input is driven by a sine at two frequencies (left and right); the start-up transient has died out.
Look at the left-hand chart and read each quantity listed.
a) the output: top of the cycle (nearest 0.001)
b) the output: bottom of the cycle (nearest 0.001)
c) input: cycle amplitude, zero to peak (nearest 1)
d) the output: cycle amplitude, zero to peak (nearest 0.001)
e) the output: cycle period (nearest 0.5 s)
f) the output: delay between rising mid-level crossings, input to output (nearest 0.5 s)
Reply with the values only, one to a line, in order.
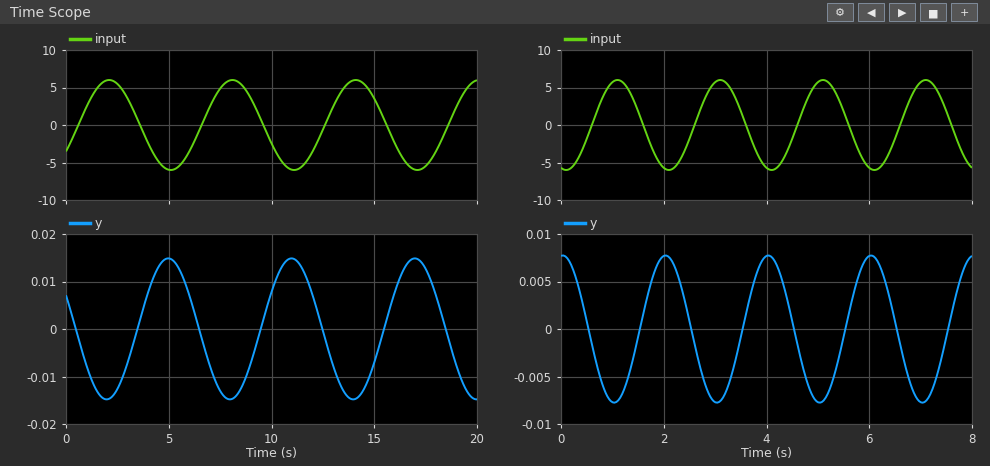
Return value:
0.015
-0.015
6
0.015
6.0 s
3.0 s
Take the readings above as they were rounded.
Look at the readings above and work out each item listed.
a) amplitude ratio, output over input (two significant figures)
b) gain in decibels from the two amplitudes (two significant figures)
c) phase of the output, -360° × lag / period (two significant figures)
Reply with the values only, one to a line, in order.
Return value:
0.0025
-52 dB
-180°
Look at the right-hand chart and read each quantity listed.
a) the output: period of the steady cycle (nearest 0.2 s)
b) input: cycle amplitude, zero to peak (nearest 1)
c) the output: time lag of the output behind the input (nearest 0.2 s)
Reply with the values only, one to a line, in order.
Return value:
2.0 s
6
1.0 s
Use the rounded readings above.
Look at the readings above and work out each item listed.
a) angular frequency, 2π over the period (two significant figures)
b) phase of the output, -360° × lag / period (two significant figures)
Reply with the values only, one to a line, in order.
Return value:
3.1 rad/s
-180°
